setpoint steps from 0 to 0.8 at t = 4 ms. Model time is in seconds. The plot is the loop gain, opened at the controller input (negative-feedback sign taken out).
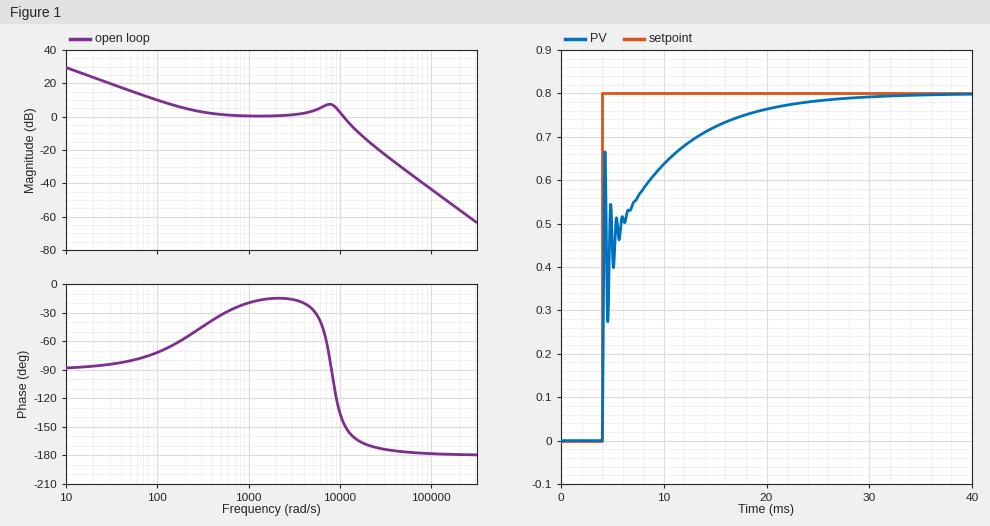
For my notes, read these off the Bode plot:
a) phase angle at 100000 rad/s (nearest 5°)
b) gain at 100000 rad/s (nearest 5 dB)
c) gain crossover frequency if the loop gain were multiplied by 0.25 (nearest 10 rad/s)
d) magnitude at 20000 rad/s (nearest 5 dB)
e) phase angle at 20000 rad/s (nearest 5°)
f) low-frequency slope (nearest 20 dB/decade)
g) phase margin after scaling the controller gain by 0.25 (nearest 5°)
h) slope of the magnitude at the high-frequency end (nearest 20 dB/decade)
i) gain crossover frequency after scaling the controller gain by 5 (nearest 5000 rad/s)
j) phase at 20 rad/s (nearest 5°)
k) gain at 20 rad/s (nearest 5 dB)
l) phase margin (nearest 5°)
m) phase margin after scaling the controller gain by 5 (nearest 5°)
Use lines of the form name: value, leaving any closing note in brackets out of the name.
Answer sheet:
phase angle at 100000 rad/s: -180°
gain at 100000 rad/s: -45 dB
gain crossover frequency if the loop gain were multiplied by 0.25: 80 rad/s
magnitude at 20000 rad/s: -15 dB
phase angle at 20000 rad/s: -170°
low-frequency slope: -20 dB/decade
phase margin after scaling the controller gain by 0.25: 105°
slope of the magnitude at the high-frequency end: -40 dB/decade
gain crossover frequency after scaling the controller gain by 5: 20000 rad/s
phase at 20 rad/s: -85°
gain at 20 rad/s: 25 dB
phase margin: 35°
phase margin after scaling the controller gain by 5: 10°
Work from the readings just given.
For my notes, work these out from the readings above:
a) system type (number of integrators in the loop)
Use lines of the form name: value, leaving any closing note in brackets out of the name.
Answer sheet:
system type: 1
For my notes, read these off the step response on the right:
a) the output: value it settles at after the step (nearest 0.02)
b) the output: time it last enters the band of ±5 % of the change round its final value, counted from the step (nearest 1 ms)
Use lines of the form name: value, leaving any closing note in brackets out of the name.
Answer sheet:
the output: value it settles at after the step: 0.80
the output: time it last enters the band of ±5 % of the change round its final value, counted from the step: 15 ms
